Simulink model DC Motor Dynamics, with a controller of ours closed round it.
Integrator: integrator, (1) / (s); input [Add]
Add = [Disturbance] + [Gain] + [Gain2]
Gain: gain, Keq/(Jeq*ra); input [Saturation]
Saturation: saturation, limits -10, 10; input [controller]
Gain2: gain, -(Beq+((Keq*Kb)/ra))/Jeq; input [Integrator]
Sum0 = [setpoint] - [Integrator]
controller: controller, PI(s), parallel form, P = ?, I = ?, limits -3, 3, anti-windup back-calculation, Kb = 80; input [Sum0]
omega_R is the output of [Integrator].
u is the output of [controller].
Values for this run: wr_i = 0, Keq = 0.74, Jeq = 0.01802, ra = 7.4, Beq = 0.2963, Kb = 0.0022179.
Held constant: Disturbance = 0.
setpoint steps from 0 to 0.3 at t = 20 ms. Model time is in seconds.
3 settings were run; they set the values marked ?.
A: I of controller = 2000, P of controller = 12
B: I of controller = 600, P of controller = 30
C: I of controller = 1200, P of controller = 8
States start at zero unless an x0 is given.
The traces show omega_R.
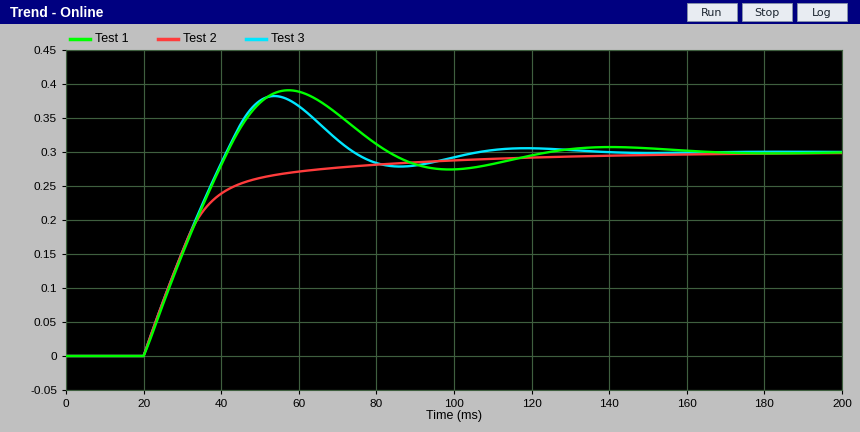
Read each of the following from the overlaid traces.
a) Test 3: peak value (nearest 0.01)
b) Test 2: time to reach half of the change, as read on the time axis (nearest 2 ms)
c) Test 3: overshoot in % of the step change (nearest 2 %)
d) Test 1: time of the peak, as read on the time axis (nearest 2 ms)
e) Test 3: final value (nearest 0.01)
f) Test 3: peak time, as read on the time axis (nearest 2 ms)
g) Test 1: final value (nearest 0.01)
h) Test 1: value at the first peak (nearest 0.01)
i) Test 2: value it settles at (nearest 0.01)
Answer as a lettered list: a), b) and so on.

a) 0.38
b) 30 ms
c) 28 %
d) 58 ms
e) 0.30
f) 54 ms
g) 0.30
h) 0.39
i) 0.30
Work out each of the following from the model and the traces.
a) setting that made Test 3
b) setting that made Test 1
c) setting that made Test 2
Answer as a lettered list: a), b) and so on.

a) A
b) C
c) B
